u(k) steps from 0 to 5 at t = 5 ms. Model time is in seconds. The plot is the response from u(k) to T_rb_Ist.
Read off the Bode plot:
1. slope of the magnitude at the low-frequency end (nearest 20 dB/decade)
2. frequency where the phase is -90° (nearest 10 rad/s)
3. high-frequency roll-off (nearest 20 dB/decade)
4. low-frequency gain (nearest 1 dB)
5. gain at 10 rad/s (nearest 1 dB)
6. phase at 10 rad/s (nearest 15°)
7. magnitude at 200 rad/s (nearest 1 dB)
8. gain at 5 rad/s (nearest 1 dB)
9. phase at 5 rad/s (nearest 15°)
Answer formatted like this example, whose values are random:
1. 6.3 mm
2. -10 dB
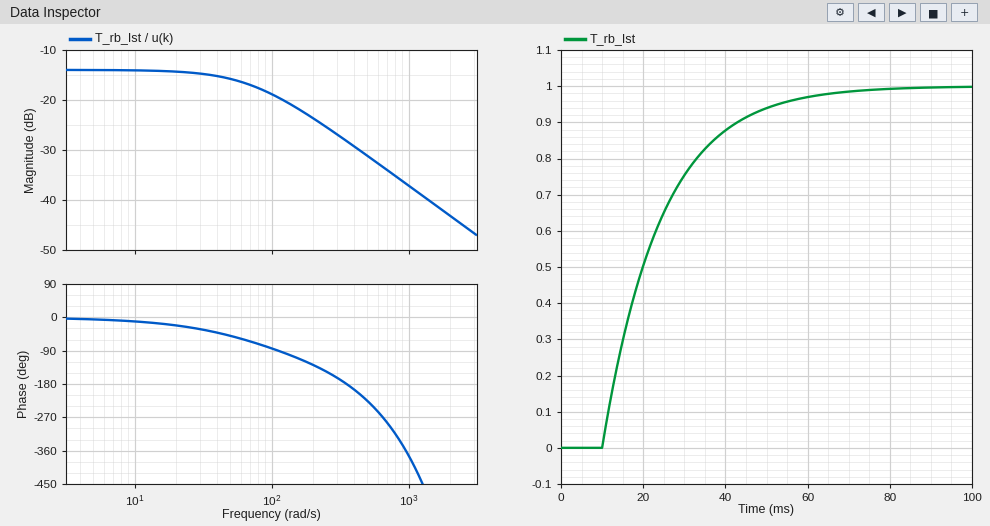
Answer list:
1. 0 dB/decade
2. 110 rad/s
3. -20 dB/decade
4. -14 dB
5. -14 dB
6. -15°
7. -24 dB
8. -14 dB
9. 0°
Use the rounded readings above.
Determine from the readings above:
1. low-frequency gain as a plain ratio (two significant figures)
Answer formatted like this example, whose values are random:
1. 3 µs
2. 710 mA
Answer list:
1. 0.20
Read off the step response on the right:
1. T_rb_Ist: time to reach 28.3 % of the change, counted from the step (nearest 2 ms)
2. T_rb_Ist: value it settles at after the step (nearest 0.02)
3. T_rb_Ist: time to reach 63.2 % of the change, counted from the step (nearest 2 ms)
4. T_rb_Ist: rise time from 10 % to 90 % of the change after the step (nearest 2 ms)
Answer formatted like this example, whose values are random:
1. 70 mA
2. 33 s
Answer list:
1. 10 ms
2. 1.00
3. 20 ms
4. 32 ms
